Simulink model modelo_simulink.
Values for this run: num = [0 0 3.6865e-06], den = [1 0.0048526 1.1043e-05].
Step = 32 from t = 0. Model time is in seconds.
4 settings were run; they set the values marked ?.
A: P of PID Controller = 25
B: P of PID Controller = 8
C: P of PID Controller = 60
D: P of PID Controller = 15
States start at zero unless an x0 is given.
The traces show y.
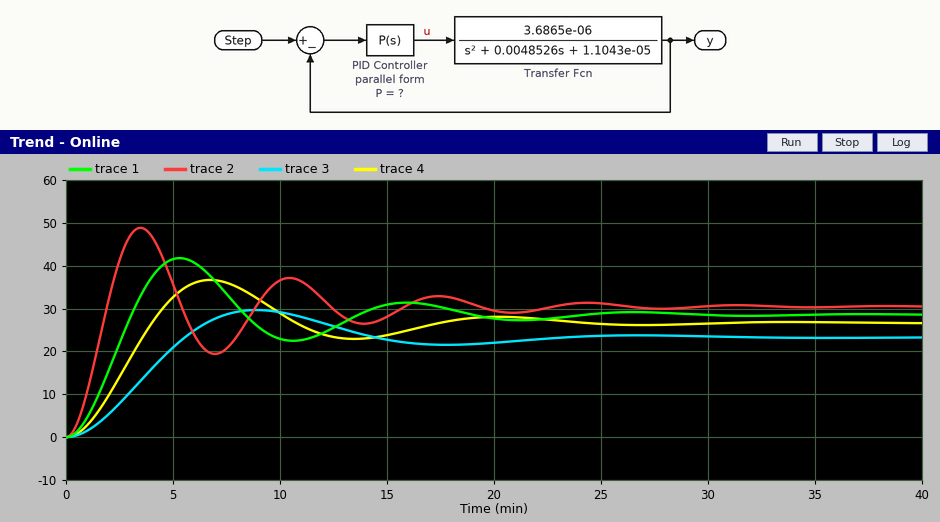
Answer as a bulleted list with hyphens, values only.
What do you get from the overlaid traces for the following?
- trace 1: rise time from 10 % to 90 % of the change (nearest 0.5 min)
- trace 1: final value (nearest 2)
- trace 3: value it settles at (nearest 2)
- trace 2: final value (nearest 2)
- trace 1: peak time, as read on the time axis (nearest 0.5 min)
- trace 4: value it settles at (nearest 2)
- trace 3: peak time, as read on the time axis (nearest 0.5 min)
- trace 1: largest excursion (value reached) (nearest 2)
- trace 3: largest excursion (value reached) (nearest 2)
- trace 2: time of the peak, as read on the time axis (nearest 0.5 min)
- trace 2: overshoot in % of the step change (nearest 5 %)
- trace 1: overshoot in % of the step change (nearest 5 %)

- 2.0 min
- 28
- 24
- 30
- 5.5 min
- 26
- 9.0 min
- 42
- 30
- 3.5 min
- 60 %
- 45 %
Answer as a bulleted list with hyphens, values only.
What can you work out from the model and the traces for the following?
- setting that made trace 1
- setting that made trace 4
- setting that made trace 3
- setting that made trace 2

- A
- D
- B
- C
